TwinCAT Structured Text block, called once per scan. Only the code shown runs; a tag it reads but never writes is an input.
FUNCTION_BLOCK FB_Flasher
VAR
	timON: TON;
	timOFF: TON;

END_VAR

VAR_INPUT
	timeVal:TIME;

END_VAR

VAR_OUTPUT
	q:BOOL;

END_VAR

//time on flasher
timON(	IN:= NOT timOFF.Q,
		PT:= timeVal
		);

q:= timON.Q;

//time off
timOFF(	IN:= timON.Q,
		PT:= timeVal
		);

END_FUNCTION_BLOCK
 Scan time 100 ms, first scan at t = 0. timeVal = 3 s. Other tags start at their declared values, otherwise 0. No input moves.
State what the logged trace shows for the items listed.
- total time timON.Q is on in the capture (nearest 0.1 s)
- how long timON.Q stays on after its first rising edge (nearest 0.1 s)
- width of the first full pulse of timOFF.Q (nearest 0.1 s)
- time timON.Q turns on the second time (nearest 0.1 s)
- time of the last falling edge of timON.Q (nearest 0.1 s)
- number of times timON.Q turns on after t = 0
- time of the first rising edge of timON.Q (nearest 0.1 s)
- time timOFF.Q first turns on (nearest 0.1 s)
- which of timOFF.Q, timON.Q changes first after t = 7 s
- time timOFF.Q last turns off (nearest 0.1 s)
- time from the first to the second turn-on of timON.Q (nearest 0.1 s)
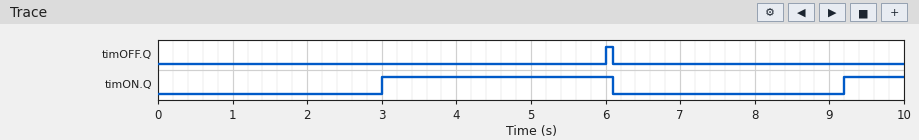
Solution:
3.9 s
3.1 s
0.1 s
9.2 s
6.1 s
2
3.0 s
6.0 s
timON.Q
6.1 s
6.2 s
